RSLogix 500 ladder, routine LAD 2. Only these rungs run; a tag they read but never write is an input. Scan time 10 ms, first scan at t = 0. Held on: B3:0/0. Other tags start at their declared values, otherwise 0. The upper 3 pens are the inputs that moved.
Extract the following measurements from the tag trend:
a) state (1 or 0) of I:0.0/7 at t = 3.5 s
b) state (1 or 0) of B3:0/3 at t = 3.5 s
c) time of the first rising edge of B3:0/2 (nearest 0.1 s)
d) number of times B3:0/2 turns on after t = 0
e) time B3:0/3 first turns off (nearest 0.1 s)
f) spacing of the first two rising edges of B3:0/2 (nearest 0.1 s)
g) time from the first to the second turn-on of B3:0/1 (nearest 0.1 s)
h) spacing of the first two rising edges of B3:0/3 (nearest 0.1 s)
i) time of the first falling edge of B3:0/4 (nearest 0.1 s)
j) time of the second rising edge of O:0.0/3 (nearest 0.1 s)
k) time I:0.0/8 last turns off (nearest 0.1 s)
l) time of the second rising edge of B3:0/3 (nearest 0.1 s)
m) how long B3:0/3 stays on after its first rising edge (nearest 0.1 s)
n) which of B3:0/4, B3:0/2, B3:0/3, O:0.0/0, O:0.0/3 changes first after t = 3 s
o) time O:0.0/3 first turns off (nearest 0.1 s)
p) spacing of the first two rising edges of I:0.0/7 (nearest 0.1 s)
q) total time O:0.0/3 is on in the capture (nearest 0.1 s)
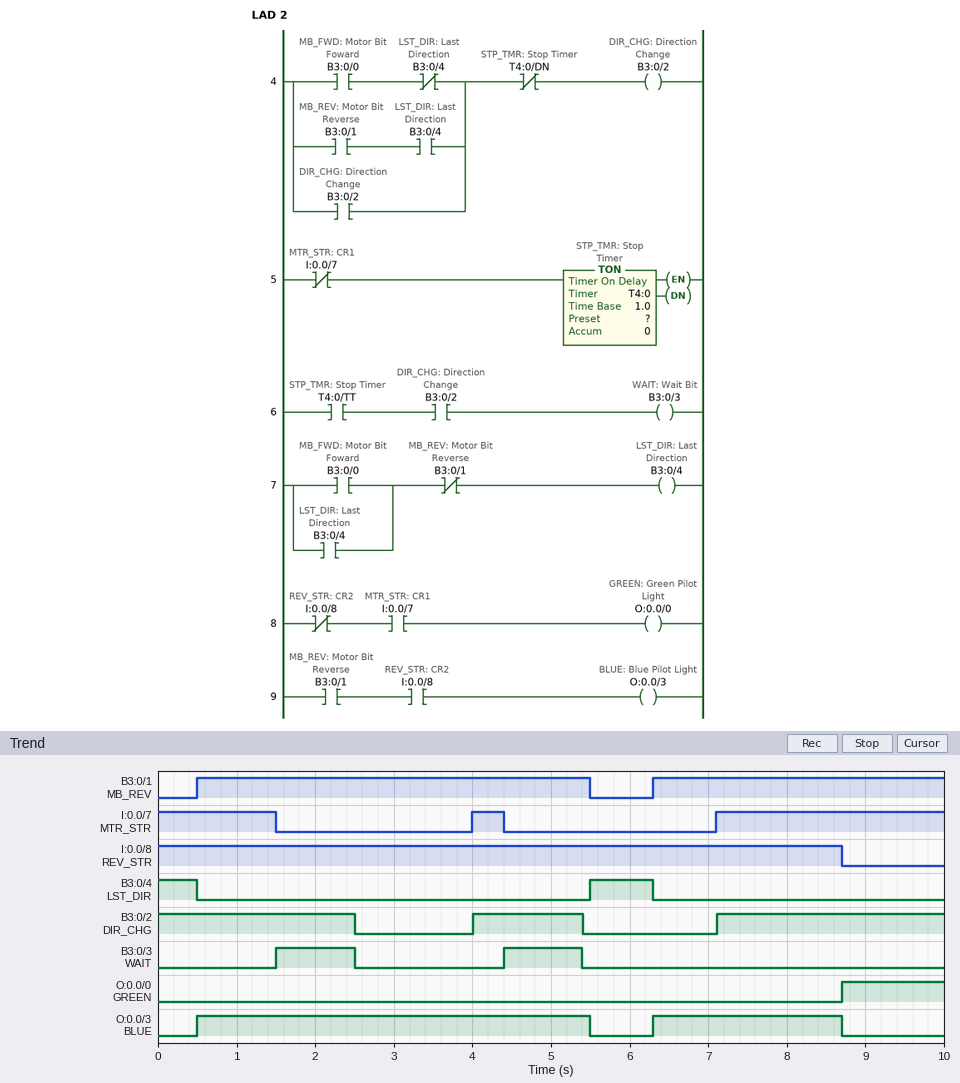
0
0
4.0 s
2
2.5 s
3.1 s
5.8 s
2.9 s
0.5 s
6.3 s
8.7 s
4.4 s
1.0 s
B3:0/2
5.5 s
3.1 s
7.4 s
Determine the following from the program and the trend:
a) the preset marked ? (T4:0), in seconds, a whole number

1 s
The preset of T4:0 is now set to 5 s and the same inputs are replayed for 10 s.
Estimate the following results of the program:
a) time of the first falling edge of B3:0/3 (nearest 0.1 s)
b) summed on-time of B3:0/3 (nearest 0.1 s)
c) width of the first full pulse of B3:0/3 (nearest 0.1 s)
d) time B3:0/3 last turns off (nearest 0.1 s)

4.0 s
5.2 s
2.5 s
7.1 s
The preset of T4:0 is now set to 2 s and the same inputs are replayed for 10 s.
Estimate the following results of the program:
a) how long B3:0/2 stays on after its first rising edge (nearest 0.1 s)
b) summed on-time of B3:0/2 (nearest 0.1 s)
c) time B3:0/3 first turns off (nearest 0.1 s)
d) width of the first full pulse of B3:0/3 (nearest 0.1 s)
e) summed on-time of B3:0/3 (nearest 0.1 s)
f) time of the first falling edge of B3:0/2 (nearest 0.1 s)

2.4 s
8.8 s
3.5 s
2.0 s
4.0 s
3.5 s
